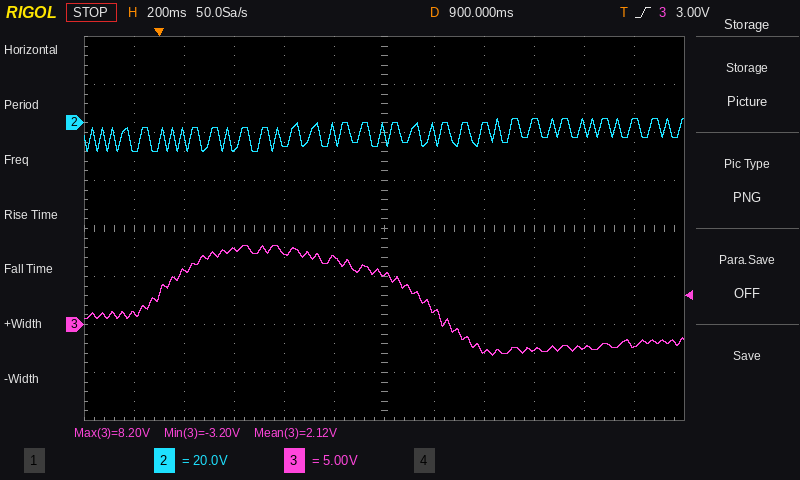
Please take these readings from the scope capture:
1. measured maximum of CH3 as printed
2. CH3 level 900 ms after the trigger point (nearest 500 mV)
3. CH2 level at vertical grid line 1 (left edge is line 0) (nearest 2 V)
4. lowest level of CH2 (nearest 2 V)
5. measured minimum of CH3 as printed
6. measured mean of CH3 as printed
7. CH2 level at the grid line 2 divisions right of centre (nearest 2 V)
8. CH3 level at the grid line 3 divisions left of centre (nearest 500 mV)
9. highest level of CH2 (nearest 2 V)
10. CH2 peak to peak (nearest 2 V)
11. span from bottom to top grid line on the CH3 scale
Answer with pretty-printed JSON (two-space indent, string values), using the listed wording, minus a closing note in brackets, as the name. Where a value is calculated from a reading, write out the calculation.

{
  "measured maximum of CH3 as printed": "8.20 V",
  "CH3 level 900 ms after the trigger point": "5.0 V",
  "CH2 level at vertical grid line 1 (left edge is line 0)": "-10 V",
  "lowest level of CH2": "-12 V",
  "measured minimum of CH3 as printed": "-3.20 V",
  "measured mean of CH3 as printed": "2.12 V",
  "CH2 level at the grid line 2 divisions right of centre": "-2 V",
  "CH3 level at the grid line 3 divisions left of centre": "8.0 V",
  "highest level of CH2": "2 V",
  "CH2 peak to peak": "2 V − (-12 V) = 14 V",
  "span from bottom to top grid line on the CH3 scale": "40 V"
}
